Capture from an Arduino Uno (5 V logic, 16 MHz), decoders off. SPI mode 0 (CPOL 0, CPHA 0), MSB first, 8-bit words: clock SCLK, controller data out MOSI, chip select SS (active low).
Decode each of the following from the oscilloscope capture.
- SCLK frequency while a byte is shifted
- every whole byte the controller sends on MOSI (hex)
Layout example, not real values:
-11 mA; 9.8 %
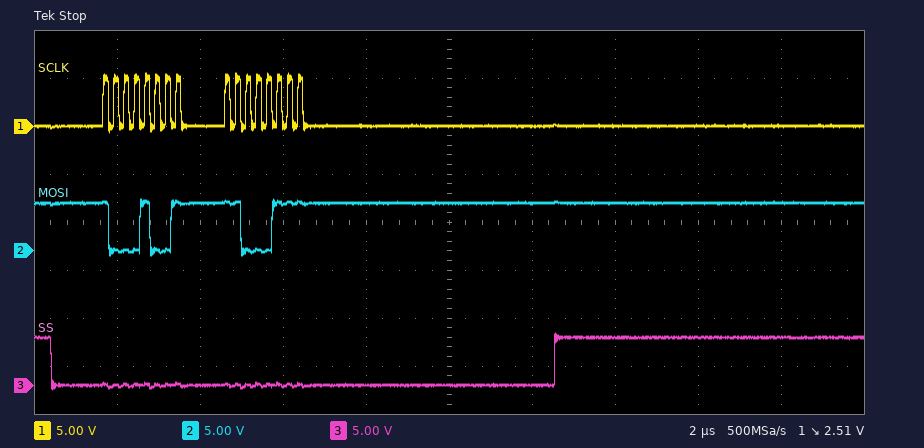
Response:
4 MHz; 0x89 0xC7
